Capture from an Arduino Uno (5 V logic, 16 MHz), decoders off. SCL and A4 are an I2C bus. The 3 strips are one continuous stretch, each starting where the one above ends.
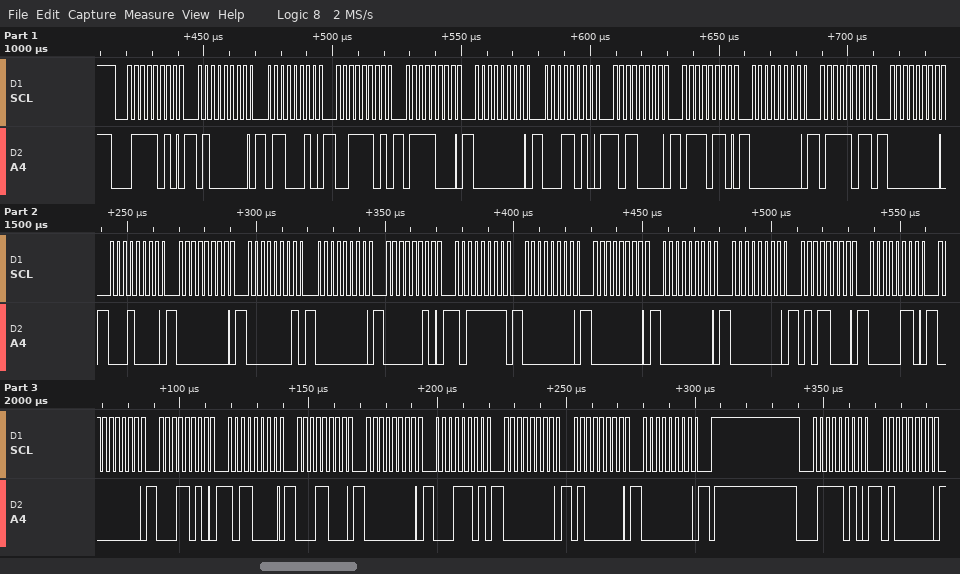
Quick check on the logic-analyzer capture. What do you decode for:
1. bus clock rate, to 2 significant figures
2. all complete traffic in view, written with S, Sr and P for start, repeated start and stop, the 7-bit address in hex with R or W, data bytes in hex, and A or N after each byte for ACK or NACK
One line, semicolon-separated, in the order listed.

400 kHz; S 3DW A 40 A 62 A 3D A 78 A 00 A 1A A B0 A 76 A 00 A 7B A 00 A 10 A 00 A 01 A 00 A 02 A BF A 00 A 00 A 00 A 00 A 58 A 06 A 00 A 1A A B0 A 18 A 00 A 1D A 00 A 40 A 00 A P S 3DW A 40 A
